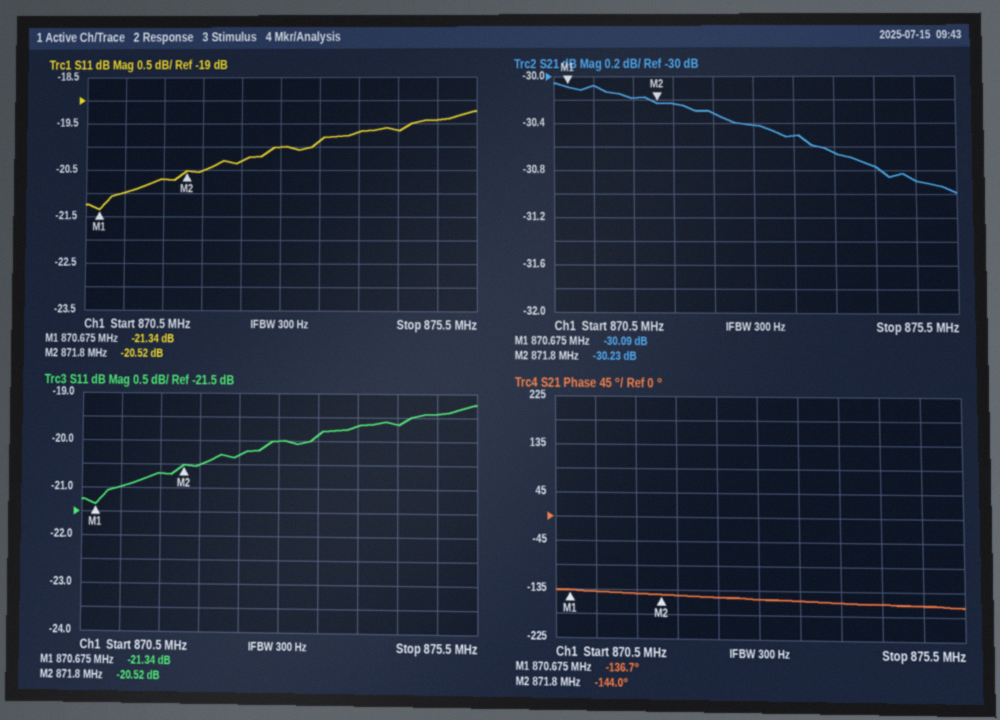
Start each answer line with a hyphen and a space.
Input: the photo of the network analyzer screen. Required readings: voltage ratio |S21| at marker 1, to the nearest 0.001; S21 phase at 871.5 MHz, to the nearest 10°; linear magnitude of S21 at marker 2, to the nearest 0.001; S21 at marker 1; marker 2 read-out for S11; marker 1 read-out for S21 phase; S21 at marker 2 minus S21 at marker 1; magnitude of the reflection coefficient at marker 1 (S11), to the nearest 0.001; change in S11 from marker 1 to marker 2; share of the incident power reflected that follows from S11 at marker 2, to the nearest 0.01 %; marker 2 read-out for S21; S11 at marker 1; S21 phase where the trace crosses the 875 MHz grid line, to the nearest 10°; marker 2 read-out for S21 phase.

- 0.031
- -140°
- 0.031
- -30.09 dB
- -20.52 dB
- -136.7°
- -0.14 dB
- 0.086
- 0.82 dB
- 0.89 %
- -30.23 dB
- -21.34 dB
- -160°
- -144.0°
